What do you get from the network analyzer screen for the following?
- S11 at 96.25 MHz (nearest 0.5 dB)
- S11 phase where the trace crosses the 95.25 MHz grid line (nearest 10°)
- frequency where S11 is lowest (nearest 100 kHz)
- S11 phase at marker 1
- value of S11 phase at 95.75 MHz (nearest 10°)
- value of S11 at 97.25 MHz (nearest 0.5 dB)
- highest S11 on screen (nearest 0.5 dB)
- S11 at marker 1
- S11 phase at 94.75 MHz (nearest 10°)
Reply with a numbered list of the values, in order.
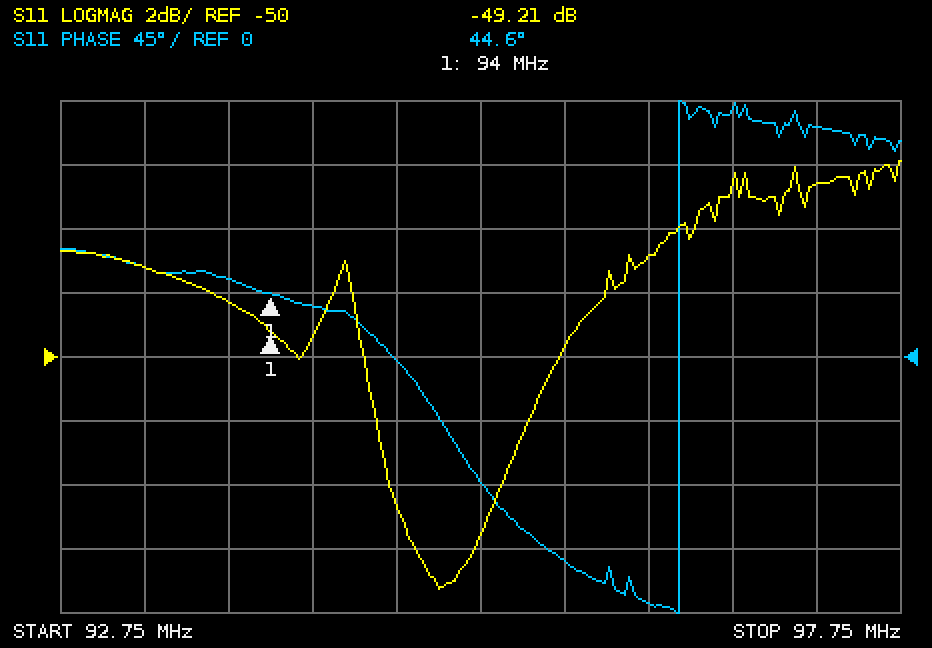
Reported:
1. -47.0 dB
2. -90°
3. 95.0 MHz
4. 44.6°
5. -140°
6. -44.5 dB
7. -44.0 dB
8. -49.21 dB
9. 0°
